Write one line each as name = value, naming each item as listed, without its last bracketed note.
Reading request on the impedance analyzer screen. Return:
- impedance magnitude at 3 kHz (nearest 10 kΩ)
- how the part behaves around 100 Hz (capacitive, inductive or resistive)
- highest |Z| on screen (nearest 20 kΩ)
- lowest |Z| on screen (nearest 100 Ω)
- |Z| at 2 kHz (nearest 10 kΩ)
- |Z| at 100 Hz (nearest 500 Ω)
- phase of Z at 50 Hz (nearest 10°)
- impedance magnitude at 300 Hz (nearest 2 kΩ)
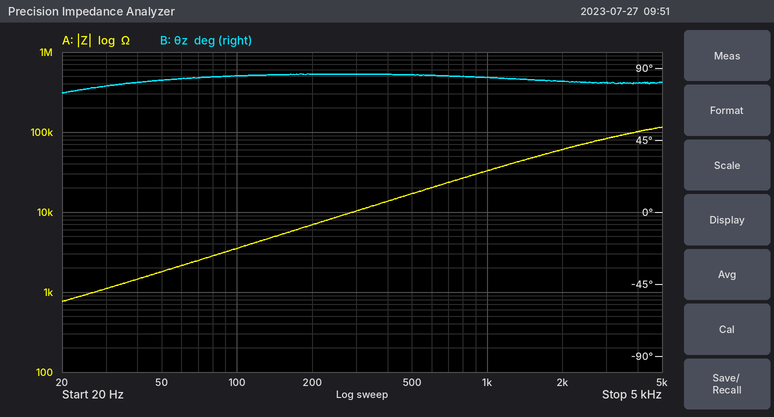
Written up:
impedance magnitude at 3 kHz = 80 kΩ
how the part behaves around 100 Hz = inductive
highest |Z| on screen = 120 kΩ
lowest |Z| on screen = 800 Ω
|Z| at 2 kHz = 60 kΩ
|Z| at 100 Hz = 3.5 kΩ
phase of Z at 50 Hz = 80°
impedance magnitude at 300 Hz = 10 kΩ
